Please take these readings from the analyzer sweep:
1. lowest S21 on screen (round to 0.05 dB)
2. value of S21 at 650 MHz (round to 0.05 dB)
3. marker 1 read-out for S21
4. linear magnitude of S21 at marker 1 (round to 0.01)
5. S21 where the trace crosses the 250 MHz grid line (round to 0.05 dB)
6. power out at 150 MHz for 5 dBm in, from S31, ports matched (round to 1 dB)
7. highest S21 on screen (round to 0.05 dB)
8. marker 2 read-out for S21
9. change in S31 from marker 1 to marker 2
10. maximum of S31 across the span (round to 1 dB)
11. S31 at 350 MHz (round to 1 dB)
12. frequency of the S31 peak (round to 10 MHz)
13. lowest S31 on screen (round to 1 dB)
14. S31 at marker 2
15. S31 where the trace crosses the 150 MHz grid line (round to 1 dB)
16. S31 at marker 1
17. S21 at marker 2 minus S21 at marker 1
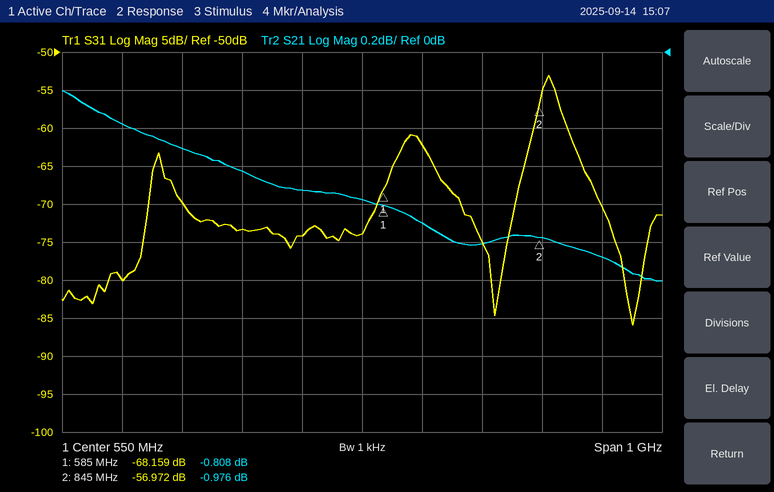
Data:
-1.20 dB
-0.90 dB
-0.808 dB
0.91
-0.50 dB
-75 dBm
-0.20 dB
-0.976 dB
11.187 dB
-53 dB
-73 dB
860 MHz
-86 dB
-56.972 dB
-80 dB
-68.159 dB
-0.168 dB
